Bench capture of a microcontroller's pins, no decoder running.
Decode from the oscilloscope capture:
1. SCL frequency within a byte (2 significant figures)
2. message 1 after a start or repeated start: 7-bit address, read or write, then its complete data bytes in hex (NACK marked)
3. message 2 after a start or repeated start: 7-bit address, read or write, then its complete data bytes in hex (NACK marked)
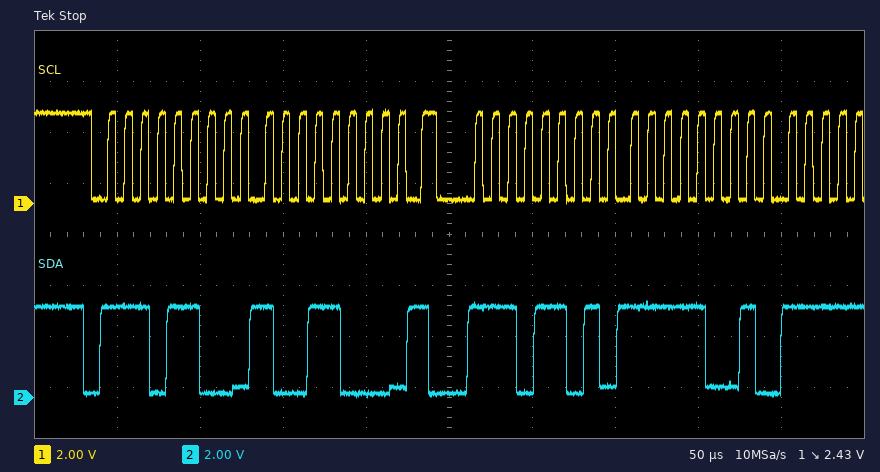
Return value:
100 kHz
0x76 write: 98
0x76 read: F9
